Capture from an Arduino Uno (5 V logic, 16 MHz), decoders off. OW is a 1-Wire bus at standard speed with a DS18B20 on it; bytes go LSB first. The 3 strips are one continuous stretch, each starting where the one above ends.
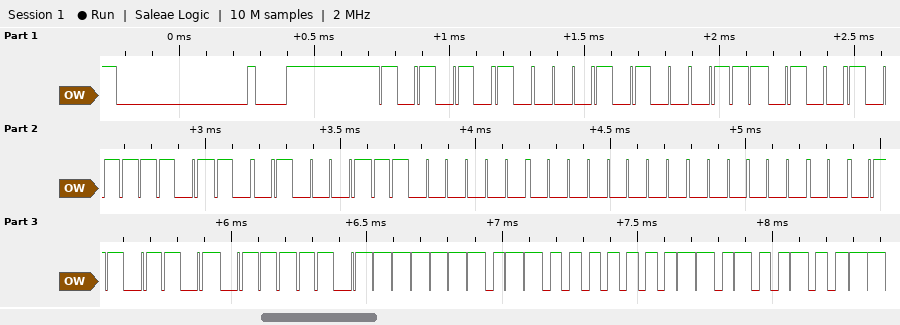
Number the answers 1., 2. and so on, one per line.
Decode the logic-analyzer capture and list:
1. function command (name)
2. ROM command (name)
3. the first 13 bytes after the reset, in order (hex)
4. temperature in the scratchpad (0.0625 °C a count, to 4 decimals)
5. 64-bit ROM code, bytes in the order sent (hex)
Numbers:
1. Read Scratchpad
2. Match ROM
3. 55 28 2E BD 89 03 00 00 B6 BE BF 01 4B
4. 27.9375 °C
5. 28 2E BD 89 03 00 00 B6
